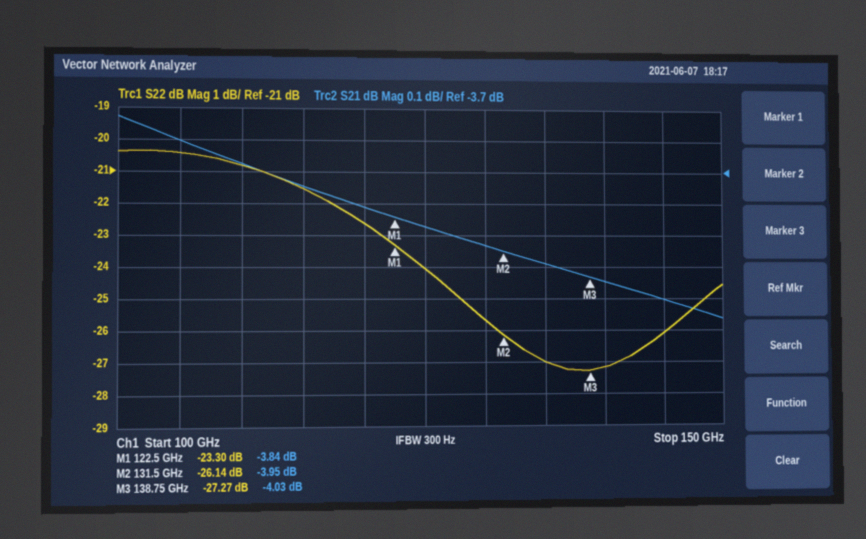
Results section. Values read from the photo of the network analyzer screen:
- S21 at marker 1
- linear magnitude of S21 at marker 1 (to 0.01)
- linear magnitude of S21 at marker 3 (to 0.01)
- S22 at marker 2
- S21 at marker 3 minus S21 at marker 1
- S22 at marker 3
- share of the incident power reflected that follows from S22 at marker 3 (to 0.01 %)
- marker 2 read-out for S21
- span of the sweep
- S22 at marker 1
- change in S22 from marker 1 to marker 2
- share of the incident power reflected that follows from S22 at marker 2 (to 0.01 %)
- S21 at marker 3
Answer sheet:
-3.84 dB
0.64
0.63
-26.14 dB
-0.19 dB
-27.27 dB
0.19 %
-3.95 dB
50 GHz
-23.30 dB
-2.84 dB
0.24 %
-4.03 dB
